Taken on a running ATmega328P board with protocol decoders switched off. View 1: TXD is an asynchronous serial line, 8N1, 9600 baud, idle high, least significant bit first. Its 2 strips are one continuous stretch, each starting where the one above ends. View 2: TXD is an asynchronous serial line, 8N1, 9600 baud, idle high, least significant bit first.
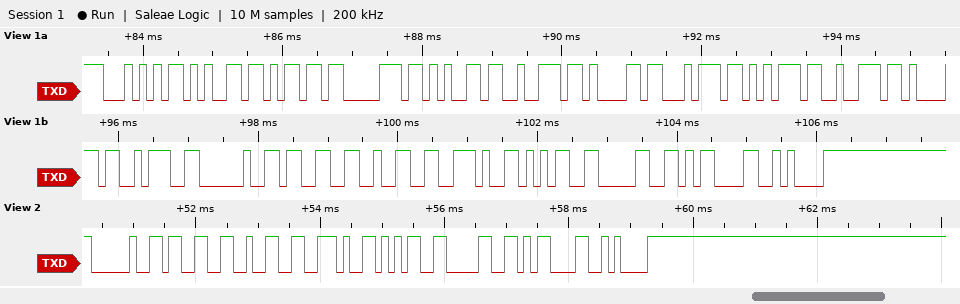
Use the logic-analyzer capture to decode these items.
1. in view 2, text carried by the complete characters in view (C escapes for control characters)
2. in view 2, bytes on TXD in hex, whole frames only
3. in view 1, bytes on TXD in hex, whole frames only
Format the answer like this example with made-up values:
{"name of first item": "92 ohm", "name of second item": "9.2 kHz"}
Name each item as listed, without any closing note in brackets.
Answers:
{"in view 2, text carried by the complete characters in view": "\" 32.50\\r\\n\"", "in view 2, bytes on TXD in hex, whole frames only": "0x20 0x33 0x32 0x2E 0x35 0x30 0x0D 0x0A", "in view 1, bytes on TXD in hex, whole frames only": "54 65 6D 70 65 72 61 74 75 72 61 3A 20 33 32 2E 35 30 0D 0A"}
